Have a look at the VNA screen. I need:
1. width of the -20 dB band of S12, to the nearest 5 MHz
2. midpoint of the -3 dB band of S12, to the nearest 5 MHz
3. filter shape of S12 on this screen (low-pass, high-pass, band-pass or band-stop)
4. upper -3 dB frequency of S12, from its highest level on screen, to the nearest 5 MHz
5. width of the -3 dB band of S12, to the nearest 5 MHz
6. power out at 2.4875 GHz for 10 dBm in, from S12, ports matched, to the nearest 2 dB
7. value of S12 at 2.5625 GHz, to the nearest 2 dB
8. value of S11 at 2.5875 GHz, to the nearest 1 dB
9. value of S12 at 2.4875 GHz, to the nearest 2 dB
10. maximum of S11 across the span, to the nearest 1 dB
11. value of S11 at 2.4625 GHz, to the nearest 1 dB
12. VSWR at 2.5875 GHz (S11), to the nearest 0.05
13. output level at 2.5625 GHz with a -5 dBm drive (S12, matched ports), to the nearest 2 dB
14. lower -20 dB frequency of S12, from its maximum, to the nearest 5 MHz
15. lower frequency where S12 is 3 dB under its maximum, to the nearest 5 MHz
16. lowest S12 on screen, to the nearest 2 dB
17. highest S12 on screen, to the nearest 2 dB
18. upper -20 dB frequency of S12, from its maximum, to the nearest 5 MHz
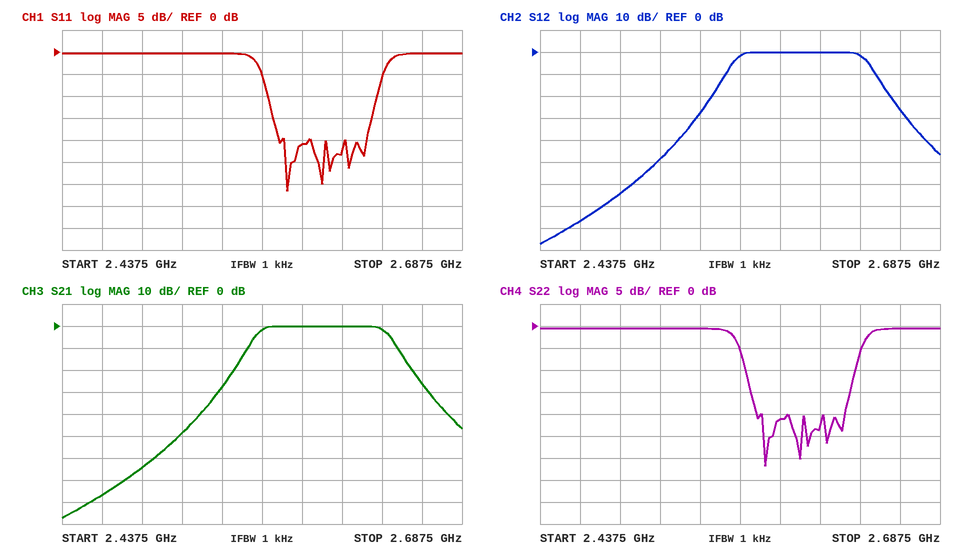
110 MHz
2.600 GHz
band-pass
2.640 GHz
80 MHz
-54 dBm
-2 dB
-21 dB
-64 dB
0 dB
0 dB
1.20
-6 dBm
2.545 GHz
2.560 GHz
-88 dB
0 dB
2.655 GHz
